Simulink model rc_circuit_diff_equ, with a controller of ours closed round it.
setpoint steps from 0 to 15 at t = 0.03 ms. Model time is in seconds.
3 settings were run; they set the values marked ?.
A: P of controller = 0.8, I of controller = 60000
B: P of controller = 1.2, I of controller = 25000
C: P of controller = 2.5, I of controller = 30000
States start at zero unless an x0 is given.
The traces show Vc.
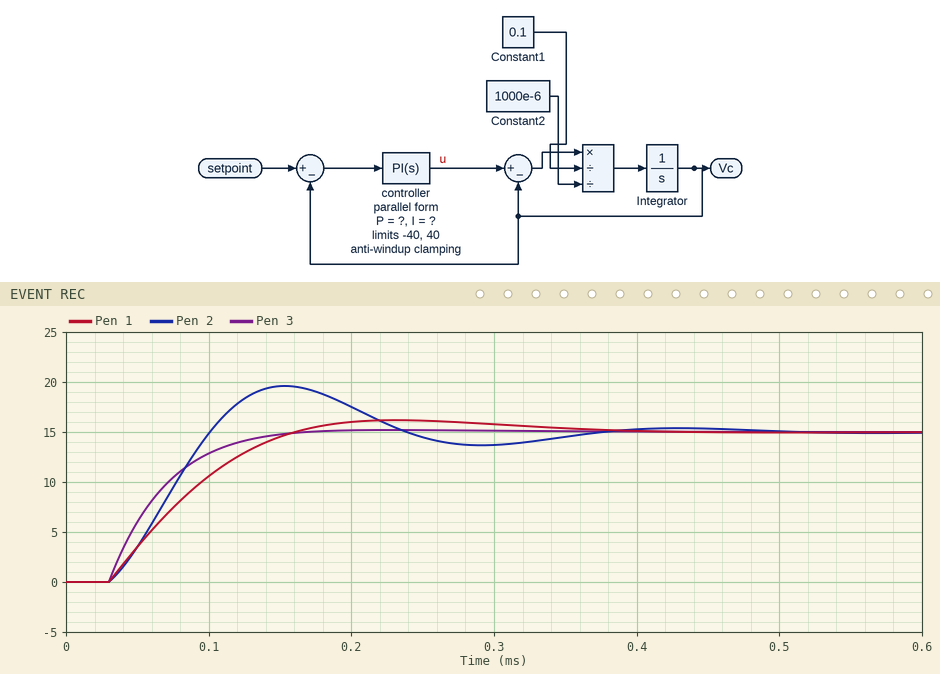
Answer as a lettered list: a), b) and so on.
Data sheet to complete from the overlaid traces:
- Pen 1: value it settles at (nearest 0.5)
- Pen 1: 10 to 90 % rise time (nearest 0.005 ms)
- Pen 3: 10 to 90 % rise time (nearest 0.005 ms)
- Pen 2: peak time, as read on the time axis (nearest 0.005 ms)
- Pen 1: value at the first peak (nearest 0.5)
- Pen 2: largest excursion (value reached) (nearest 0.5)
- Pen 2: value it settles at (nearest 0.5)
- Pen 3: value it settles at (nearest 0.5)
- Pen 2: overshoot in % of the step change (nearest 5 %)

a) 15.0
b) 0.095 ms
c) 0.075 ms
d) 0.155 ms
e) 16.0
f) 19.5
g) 15.0
h) 15.0
i) 30 %
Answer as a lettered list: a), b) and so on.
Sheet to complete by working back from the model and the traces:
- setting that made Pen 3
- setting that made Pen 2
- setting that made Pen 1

a) C
b) A
c) B
